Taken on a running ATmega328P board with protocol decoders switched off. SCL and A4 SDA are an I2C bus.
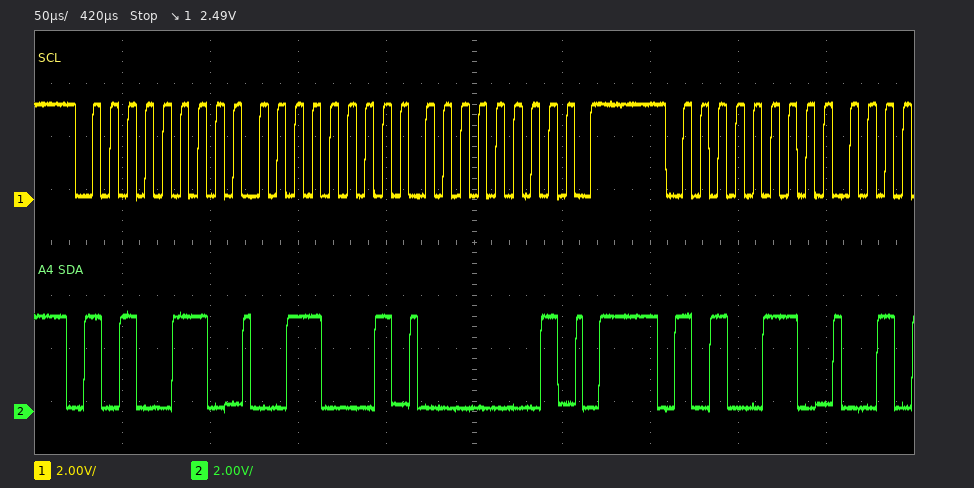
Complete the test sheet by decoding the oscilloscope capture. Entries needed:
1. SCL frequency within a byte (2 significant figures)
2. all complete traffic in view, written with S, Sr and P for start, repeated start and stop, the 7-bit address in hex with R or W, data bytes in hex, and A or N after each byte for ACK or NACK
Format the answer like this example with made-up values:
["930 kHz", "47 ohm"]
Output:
["100 kHz", "S 53W A 31 A 01 A P S 53W A"]
